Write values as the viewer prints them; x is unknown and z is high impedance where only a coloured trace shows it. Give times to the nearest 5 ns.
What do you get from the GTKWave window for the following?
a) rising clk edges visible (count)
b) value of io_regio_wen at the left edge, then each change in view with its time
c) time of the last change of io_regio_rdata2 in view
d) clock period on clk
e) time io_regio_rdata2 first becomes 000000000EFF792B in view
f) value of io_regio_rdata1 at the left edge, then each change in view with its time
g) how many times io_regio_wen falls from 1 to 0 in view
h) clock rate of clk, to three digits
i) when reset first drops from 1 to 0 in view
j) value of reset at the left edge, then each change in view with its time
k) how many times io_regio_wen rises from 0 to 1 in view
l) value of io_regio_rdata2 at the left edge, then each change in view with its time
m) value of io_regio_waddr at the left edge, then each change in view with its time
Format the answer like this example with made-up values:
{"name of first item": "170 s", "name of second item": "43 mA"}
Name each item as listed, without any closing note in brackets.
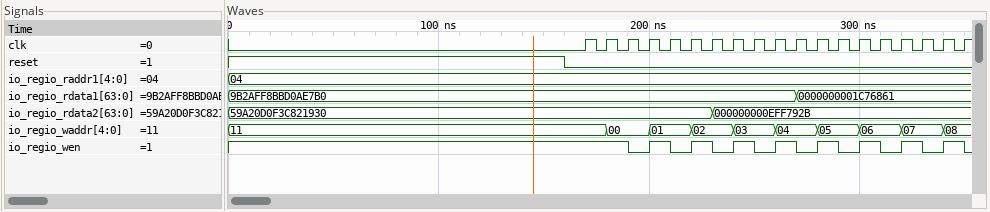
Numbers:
{"rising clk edges visible": "19", "value of io_regio_wen at the left edge, then each change in view with its time": "1, 0 at 190 ns, 1 at 200 ns, 0 at 210 ns, 1 at 220 ns, 0 at 230 ns, 1 at 240 ns, 0 at 250 ns, 1 at 260 ns, 0 at 270 ns, 1 at 280 ns, 0 at 290 ns, 1 at 300 ns, 0 at 310 ns, 1 at 320 ns, 0 at 330 ns, 1 at 340 ns, 0 at 350 ns", "time of the last change of io_regio_rdata2 in view": "230 ns", "clock period on clk": "10 ns", "time io_regio_rdata2 first becomes 000000000EFF792B in view": "230 ns", "value of io_regio_rdata1 at the left edge, then each change in view with its time": "9B2AFF8BBD0AE7B0, 0000000001C76861 at 270 ns", "how many times io_regio_wen falls from 1 to 0 in view": "9", "clock rate of clk, to three digits": "100 MHz", "when reset first drops from 1 to 0 in view": "160 ns", "value of reset at the left edge, then each change in view with its time": "1, 0 at 160 ns", "how many times io_regio_wen rises from 0 to 1 in view": "8", "value of io_regio_rdata2 at the left edge, then each change in view with its time": "59A20D0F3C821930, 000000000EFF792B at 230 ns", "value of io_regio_waddr at the left edge, then each change in view with its time": "11, 00 at 180 ns, 01 at 200 ns, 02 at 220 ns, 03 at 240 ns, 04 at 260 ns, 05 at 280 ns, 06 at 300 ns, 07 at 320 ns, 08 at 340 ns"}
